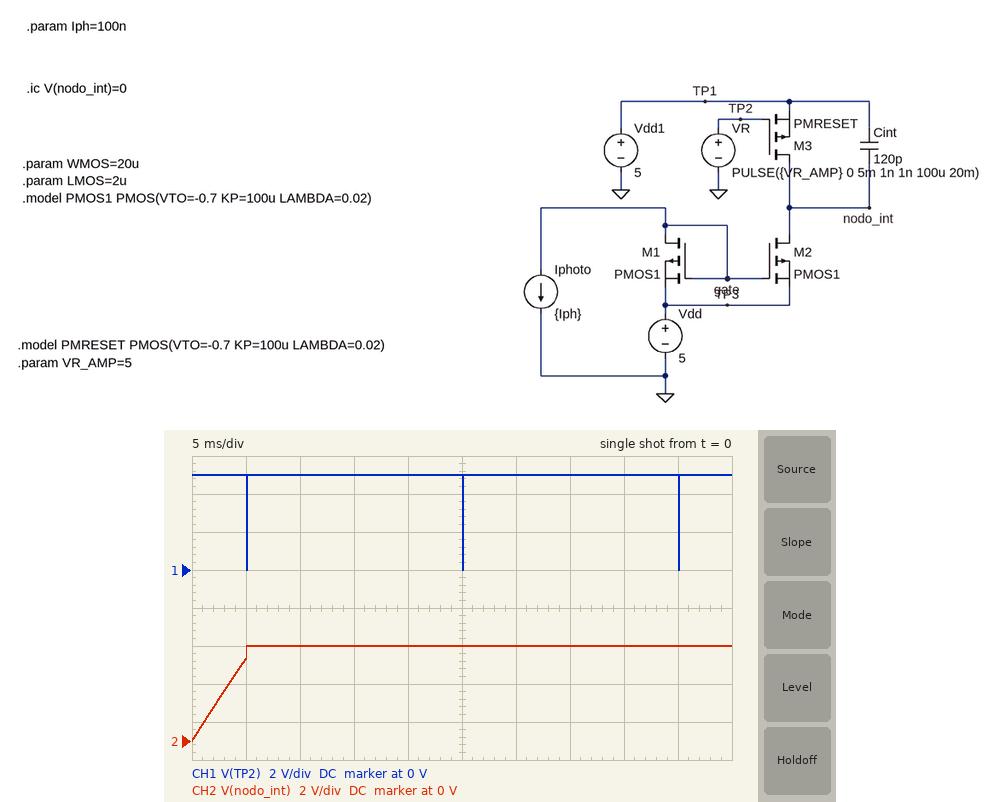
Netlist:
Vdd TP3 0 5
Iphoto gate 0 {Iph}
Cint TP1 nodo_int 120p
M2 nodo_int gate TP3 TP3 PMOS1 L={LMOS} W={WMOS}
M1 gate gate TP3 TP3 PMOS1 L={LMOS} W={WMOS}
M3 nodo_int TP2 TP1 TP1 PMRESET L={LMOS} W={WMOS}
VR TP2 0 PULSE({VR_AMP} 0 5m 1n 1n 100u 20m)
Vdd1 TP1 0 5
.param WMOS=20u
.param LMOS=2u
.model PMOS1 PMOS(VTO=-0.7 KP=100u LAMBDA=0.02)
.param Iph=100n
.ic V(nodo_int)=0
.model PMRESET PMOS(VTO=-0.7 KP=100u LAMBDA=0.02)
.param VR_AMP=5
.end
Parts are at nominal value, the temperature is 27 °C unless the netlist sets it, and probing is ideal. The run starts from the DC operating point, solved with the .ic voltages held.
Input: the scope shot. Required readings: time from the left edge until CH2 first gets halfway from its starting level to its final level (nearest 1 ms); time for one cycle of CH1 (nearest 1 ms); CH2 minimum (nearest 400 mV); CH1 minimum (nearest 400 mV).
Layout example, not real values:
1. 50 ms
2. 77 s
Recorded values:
1. 3 ms
2. 20 ms
3. 0 V
4. 0 V
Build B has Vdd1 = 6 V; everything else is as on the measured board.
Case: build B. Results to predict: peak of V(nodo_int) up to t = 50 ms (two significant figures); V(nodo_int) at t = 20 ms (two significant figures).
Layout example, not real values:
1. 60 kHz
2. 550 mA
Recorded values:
1. 5.7 V
2. 5.3 V
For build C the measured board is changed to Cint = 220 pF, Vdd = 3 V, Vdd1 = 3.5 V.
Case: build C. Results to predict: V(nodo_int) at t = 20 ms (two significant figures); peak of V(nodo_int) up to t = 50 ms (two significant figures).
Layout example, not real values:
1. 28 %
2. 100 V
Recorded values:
1. 3.0 V
2. 3.5 V
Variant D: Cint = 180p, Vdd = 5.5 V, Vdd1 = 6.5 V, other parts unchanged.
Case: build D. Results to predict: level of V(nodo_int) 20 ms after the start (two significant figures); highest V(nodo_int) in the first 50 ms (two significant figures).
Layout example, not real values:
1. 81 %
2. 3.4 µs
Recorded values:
1. 6.1 V
2. 6.2 V
